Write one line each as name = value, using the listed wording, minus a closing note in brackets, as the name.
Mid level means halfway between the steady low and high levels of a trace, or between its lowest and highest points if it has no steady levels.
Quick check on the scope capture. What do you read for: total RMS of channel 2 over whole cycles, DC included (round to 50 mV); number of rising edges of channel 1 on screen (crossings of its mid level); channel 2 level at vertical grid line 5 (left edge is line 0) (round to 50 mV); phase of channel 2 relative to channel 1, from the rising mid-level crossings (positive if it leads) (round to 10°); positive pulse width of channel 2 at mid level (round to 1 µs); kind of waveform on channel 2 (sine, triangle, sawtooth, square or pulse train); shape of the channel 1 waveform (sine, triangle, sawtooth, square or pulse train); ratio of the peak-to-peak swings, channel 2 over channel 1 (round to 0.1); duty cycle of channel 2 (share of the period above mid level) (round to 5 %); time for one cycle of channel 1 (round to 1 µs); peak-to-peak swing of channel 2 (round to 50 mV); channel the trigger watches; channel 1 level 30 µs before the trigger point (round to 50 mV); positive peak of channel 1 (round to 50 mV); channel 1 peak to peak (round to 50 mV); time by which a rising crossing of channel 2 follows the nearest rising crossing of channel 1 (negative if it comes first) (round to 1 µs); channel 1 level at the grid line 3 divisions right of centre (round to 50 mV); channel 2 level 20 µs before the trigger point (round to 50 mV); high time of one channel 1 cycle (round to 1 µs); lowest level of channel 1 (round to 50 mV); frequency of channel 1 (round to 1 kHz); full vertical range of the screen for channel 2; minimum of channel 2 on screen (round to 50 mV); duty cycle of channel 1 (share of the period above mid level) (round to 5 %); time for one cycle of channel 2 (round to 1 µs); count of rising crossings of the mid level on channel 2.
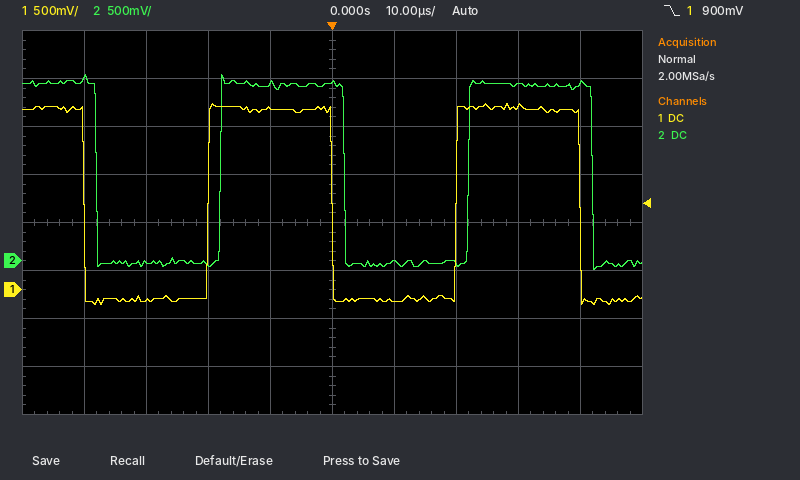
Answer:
total RMS of channel 2 over whole cycles, DC included = 1.30 V
number of rising edges of channel 1 on screen = 2
channel 2 level at vertical grid line 5 (left edge is line 0) = 1.85 V
phase of channel 2 relative to channel 1, from the rising mid-level crossings (positive if it leads) = -20°
positive pulse width of channel 2 at mid level = 20 µs
kind of waveform on channel 2 = square
shape of the channel 1 waveform = square
ratio of the peak-to-peak swings, channel 2 over channel 1 = 1.0
duty cycle of channel 2 (share of the period above mid level) = 50 %
time for one cycle of channel 1 = 40 µs
peak-to-peak swing of channel 2 = 2.05 V
channel the trigger watches = channel 1
channel 1 level 30 µs before the trigger point = -100 mV
positive peak of channel 1 = 1.95 V
channel 1 peak to peak = 2.10 V
time by which a rising crossing of channel 2 follows the nearest rising crossing of channel 1 (negative if it comes first) = +2 µs
channel 1 level at the grid line 3 divisions right of centre = 1.90 V
channel 2 level 20 µs before the trigger point = -50 mV
high time of one channel 1 cycle = 20 µs
lowest level of channel 1 = -150 mV
frequency of channel 1 = 25 kHz
full vertical range of the screen for channel 2 = 4 V
minimum of channel 2 on screen = -100 mV
duty cycle of channel 1 (share of the period above mid level) = 50 %
time for one cycle of channel 2 = 40 µs
count of rising crossings of the mid level on channel 2 = 2
